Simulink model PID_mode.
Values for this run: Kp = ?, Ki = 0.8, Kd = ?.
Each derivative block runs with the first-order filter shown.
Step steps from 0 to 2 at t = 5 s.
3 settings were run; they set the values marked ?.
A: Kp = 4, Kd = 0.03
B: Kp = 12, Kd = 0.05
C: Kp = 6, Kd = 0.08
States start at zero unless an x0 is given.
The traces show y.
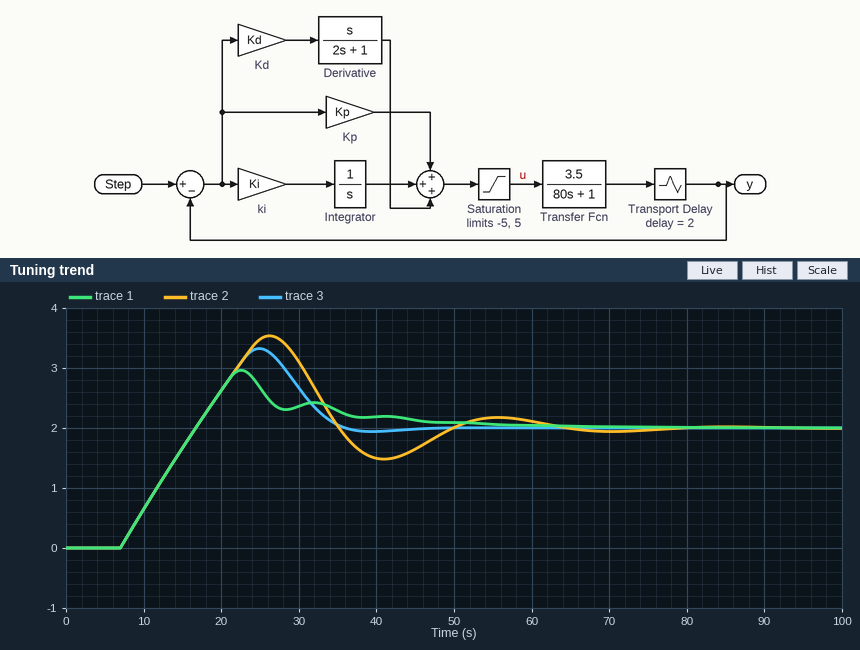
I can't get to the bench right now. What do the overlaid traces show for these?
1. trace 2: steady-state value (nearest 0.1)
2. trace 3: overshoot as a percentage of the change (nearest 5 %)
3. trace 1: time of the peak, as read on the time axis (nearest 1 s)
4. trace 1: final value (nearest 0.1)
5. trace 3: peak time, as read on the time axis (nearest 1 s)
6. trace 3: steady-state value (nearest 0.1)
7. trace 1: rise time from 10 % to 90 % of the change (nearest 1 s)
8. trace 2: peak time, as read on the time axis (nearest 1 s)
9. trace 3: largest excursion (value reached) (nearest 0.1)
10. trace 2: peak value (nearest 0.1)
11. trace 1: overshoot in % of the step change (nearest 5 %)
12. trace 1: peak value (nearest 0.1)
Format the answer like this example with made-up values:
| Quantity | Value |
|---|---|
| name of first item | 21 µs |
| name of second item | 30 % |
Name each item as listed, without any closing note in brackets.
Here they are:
| Quantity | Value |
|---|---|
| trace 2: steady-state value | 2.0 |
| trace 3: overshoot as a percentage of the change | 65 % |
| trace 1: time of the peak, as read on the time axis | 23 s |
| trace 1: final value | 2.0 |
| trace 3: peak time, as read on the time axis | 25 s |
| trace 3: steady-state value | 2.0 |
| trace 1: rise time from 10 % to 90 % of the change | 8 s |
| trace 2: peak time, as read on the time axis | 26 s |
| trace 3: largest excursion (value reached) | 3.3 |
| trace 2: peak value | 3.5 |
| trace 1: overshoot in % of the step change | 50 % |
| trace 1: peak value | 3.0 |
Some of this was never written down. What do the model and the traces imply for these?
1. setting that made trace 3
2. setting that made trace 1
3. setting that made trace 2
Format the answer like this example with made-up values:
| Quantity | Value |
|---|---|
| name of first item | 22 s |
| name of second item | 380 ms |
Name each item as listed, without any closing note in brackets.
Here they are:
| Quantity | Value |
|---|---|
| setting that made trace 3 | C |
| setting that made trace 1 | B |
| setting that made trace 2 | A |
